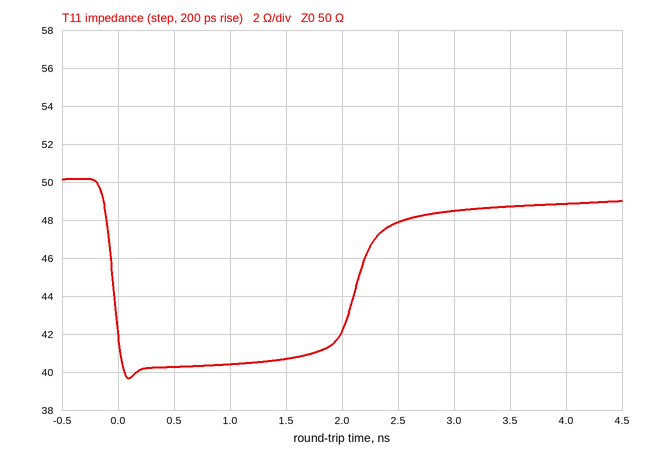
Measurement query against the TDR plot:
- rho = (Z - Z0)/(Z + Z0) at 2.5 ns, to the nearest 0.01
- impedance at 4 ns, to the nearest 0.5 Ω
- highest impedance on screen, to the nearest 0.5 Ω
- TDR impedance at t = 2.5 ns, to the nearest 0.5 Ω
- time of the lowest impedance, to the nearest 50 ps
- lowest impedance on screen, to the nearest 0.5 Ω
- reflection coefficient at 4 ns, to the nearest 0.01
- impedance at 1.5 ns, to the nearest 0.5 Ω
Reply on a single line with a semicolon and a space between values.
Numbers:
-0.02; 49.0 Ω; 50.0 Ω; 48.0 Ω; 100 ps; 39.5 Ω; -0.01; 40.5 Ω
